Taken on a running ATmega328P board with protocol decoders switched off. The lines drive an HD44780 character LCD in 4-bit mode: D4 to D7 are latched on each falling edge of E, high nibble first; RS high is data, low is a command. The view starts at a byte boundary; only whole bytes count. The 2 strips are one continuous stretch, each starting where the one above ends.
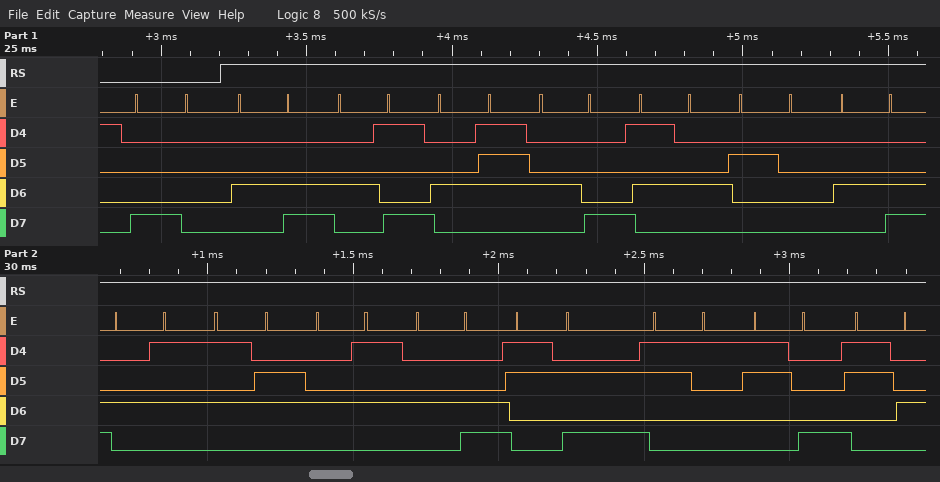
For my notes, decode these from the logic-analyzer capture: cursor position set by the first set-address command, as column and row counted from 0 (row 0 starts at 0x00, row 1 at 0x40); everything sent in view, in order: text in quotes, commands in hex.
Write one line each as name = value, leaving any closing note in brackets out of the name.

cursor position set by the first set-address command, as column and row counted from 0 = column 0, row 0
everything sent in view, in order: text in quotes, commands in hex = 0x80 "LIGHT LEVEL:184"
